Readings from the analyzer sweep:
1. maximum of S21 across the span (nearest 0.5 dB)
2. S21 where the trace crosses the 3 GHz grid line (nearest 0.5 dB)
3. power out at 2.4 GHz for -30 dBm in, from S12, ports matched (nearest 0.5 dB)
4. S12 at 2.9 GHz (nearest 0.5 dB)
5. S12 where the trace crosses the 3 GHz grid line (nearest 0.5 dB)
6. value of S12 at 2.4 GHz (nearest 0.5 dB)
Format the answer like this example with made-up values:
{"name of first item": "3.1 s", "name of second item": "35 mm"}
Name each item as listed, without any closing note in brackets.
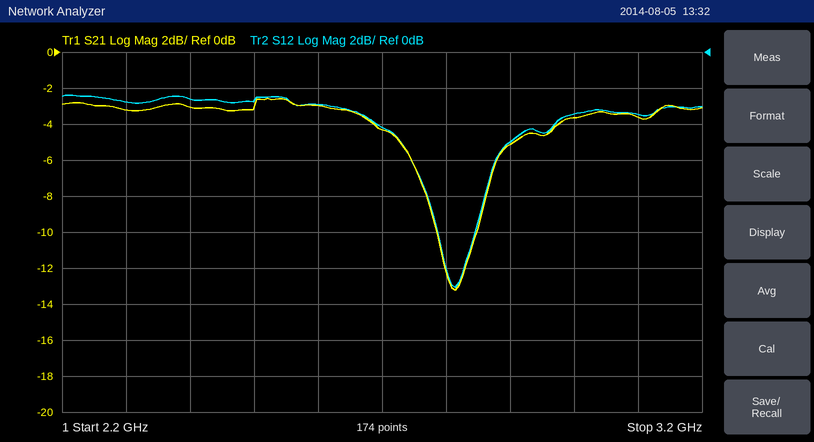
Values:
{"maximum of S21 across the span": "-2.5 dB", "S21 where the trace crosses the 3 GHz grid line": "-3.5 dB", "power out at 2.4 GHz for -30 dBm in, from S12, ports matched": "-32.5 dBm", "S12 at 2.9 GHz": "-5.0 dB", "S12 where the trace crosses the 3 GHz grid line": "-3.5 dB", "value of S12 at 2.4 GHz": "-2.5 dB"}
